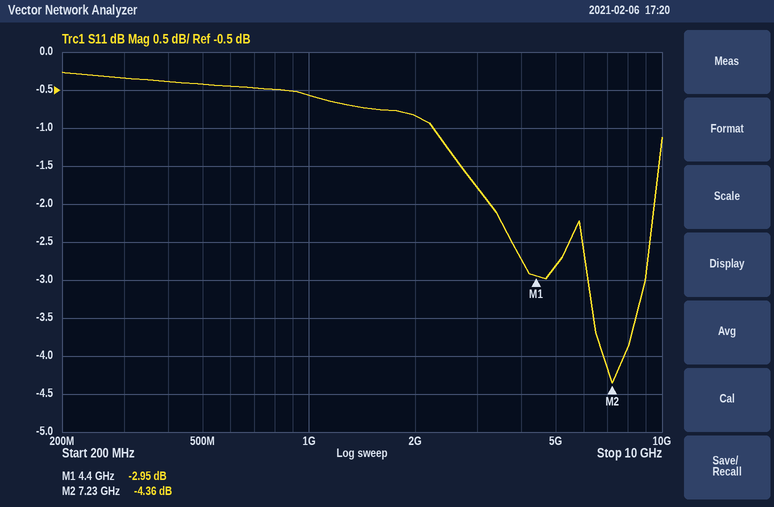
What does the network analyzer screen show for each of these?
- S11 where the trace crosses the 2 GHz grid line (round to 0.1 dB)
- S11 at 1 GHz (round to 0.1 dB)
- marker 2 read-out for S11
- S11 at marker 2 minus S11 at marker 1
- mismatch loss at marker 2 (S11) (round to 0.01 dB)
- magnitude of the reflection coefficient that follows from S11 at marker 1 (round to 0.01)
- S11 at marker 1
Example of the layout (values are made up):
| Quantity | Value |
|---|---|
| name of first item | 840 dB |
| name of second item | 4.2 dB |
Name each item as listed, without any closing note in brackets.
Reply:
| Quantity | Value |
|---|---|
| S11 where the trace crosses the 2 GHz grid line | -0.8 dB |
| S11 at 1 GHz | -0.6 dB |
| marker 2 read-out for S11 | -4.36 dB |
| S11 at marker 2 minus S11 at marker 1 | -1.41 dB |
| mismatch loss at marker 2 (S11) | 1.98 dB |
| magnitude of the reflection coefficient that follows from S11 at marker 1 | 0.71 |
| S11 at marker 1 | -2.95 dB |
